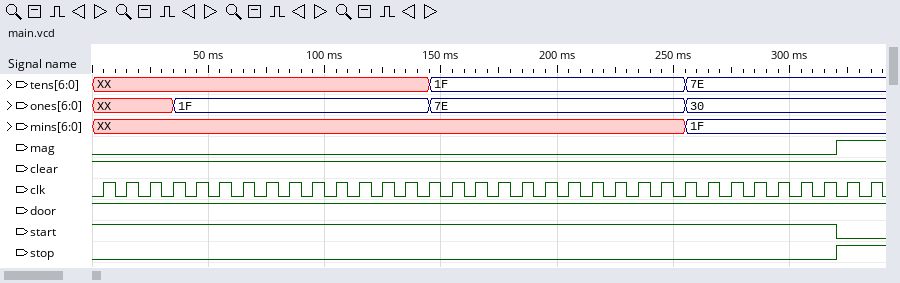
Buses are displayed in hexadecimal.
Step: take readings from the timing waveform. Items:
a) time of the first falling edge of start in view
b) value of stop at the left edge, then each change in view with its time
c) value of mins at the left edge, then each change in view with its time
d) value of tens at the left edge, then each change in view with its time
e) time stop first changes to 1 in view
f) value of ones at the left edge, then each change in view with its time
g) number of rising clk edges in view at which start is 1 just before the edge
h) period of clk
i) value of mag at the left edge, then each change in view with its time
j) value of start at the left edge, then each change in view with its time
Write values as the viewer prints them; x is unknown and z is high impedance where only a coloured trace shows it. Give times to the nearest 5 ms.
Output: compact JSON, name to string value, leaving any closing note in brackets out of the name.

{"time of the first falling edge of start in view": "320 ms", "value of stop at the left edge, then each change in view with its time": "0, 1 at 320 ms", "value of mins at the left edge, then each change in view with its time": "XX, 1F at 255 ms", "value of tens at the left edge, then each change in view with its time": "XX, 1F at 145 ms, 7E at 255 ms", "time stop first changes to 1 in view": "320 ms", "value of ones at the left edge, then each change in view with its time": "XX, 1F at 35 ms, 7E at 145 ms, 30 at 255 ms", "number of rising clk edges in view at which start is 1 just before the edge": "32", "period of clk": "10 ms", "value of mag at the left edge, then each change in view with its time": "0, 1 at 320 ms", "value of start at the left edge, then each change in view with its time": "1, 0 at 320 ms"}
